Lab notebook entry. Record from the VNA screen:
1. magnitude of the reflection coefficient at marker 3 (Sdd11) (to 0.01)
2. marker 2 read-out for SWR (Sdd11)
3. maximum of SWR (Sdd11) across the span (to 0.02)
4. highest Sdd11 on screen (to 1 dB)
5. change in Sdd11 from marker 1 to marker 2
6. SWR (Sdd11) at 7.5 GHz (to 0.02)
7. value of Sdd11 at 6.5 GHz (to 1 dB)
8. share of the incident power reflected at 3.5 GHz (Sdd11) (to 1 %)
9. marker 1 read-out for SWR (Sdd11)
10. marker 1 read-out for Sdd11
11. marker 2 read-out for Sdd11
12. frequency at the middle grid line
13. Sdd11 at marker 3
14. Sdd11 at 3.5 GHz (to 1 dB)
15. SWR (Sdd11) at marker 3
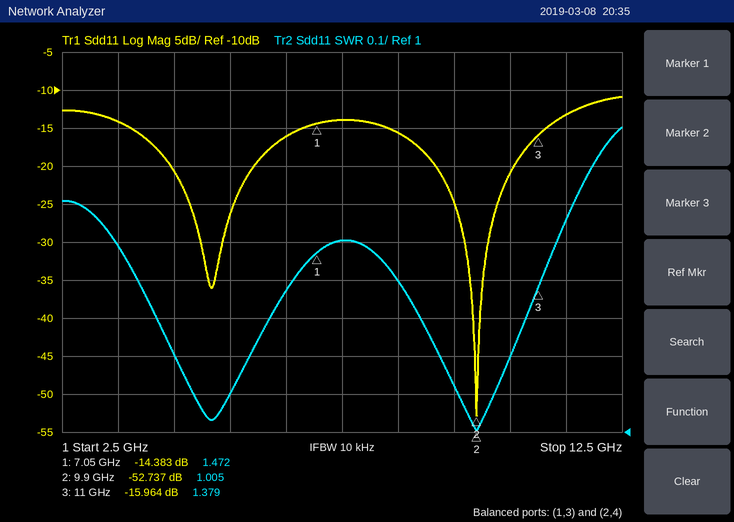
0.16
1.005
1.80
-11 dB
-38.354 dB
1.50
-16 dB
4 %
1.472
-14.383 dB
-52.737 dB
7.5 GHz
-15.964 dB
-14 dB
1.379
